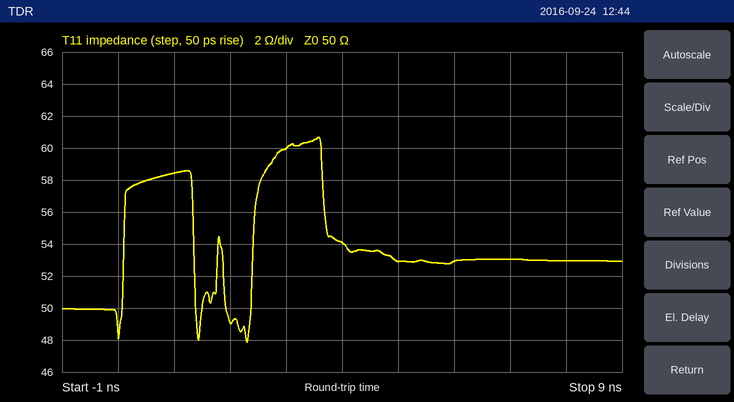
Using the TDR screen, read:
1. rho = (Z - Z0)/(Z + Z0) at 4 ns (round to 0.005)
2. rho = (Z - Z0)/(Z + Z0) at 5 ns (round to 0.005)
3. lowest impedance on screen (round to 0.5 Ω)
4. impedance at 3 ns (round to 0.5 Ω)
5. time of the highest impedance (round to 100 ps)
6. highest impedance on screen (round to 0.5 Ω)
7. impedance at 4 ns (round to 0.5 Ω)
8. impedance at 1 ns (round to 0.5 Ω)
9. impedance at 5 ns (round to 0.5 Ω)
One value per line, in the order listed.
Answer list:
+0.040
+0.030
48.0 Ω
60.0 Ω
3.6 ns
60.5 Ω
54.0 Ω
58.5 Ω
53.0 Ω
